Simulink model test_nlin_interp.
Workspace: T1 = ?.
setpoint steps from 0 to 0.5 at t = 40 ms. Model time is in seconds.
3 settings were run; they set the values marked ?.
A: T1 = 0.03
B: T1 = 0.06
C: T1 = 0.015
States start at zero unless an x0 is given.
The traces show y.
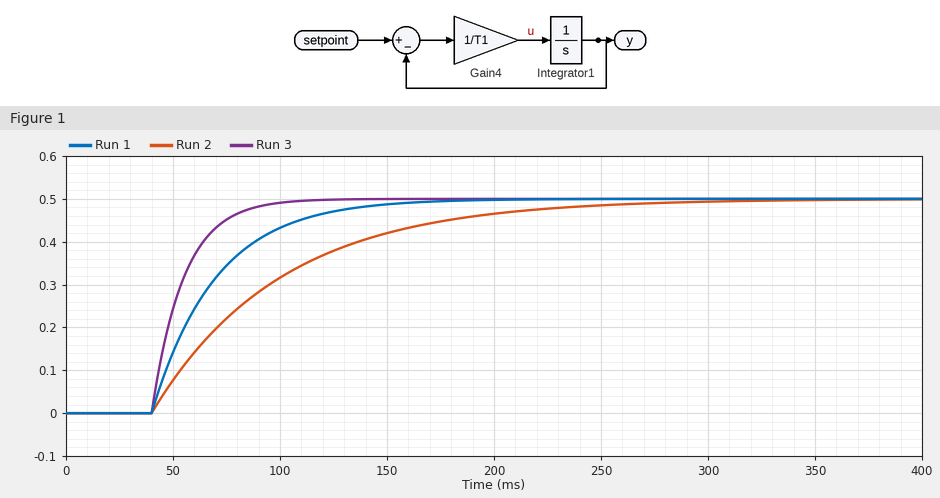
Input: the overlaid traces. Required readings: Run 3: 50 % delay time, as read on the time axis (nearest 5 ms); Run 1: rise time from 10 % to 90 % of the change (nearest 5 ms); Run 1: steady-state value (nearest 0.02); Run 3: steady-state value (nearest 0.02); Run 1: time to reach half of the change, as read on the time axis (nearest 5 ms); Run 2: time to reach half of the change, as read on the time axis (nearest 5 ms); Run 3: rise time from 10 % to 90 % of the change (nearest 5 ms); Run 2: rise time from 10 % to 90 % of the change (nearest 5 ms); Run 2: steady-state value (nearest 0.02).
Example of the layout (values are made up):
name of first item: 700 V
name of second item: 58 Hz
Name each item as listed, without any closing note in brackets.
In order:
Run 3: 50 % delay time, as read on the time axis: 50 ms
Run 1: rise time from 10 % to 90 % of the change: 65 ms
Run 1: steady-state value: 0.50
Run 3: steady-state value: 0.50
Run 1: time to reach half of the change, as read on the time axis: 60 ms
Run 2: time to reach half of the change, as read on the time axis: 80 ms
Run 3: rise time from 10 % to 90 % of the change: 35 ms
Run 2: rise time from 10 % to 90 % of the change: 130 ms
Run 2: steady-state value: 0.50
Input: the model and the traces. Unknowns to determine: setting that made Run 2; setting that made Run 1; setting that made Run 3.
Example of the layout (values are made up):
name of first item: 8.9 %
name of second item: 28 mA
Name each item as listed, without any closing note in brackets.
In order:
setting that made Run 2: B
setting that made Run 1: A
setting that made Run 3: C
